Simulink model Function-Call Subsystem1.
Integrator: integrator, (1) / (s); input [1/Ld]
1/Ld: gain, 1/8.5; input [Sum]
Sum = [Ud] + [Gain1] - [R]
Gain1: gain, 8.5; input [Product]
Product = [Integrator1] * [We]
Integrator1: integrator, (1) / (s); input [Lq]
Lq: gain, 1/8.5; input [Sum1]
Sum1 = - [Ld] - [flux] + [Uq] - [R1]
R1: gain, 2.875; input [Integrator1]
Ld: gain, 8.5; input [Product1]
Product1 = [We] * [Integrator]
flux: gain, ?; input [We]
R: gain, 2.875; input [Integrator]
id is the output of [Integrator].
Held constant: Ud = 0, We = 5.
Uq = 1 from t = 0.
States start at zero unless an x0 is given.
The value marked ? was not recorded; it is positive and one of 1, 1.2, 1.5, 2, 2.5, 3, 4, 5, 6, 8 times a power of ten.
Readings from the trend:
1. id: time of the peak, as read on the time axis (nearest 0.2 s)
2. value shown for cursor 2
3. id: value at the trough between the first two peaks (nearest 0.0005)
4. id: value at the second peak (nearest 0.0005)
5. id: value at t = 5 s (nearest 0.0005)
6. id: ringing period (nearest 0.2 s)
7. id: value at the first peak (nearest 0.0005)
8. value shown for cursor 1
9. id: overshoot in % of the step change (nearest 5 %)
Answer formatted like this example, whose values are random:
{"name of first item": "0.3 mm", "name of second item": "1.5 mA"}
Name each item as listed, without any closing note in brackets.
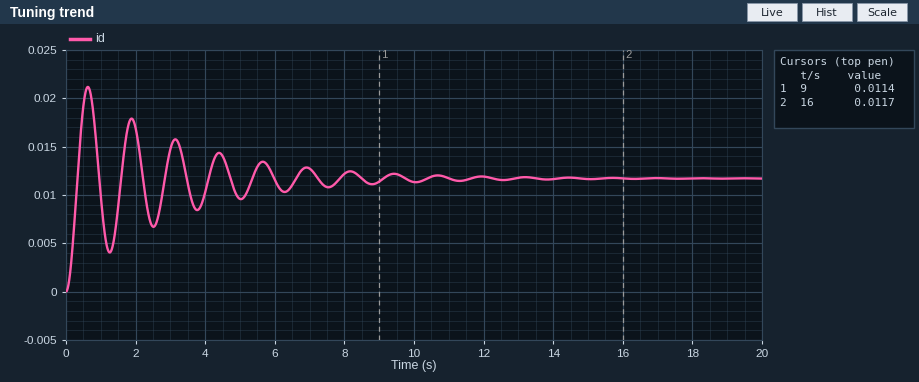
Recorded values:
{"id: time of the peak, as read on the time axis": "0.6 s", "value shown for cursor 2": "0.0117", "id: value at the trough between the first two peaks": "0.0040", "id: value at the second peak": "0.0180", "id: value at t = 5 s": "0.0095", "id: ringing period": "1.2 s", "id: value at the first peak": "0.0210", "value shown for cursor 1": "0.0114", "id: overshoot in % of the step change": "80 %"}
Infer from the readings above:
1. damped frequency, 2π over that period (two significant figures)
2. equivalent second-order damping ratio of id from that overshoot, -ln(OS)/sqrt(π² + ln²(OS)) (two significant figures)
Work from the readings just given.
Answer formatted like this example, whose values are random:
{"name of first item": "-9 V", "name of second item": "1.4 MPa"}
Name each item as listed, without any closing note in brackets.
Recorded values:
{"damped frequency, 2π over that period": "5.2 rad/s", "equivalent second-order damping ratio of id from that overshoot, -ln(OS)/sqrt(π² + ln²(OS))": "0.071"}
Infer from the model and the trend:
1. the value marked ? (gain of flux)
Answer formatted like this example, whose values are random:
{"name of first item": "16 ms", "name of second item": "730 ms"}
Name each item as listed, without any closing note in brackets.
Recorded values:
{"the value marked ?": "0.1"}
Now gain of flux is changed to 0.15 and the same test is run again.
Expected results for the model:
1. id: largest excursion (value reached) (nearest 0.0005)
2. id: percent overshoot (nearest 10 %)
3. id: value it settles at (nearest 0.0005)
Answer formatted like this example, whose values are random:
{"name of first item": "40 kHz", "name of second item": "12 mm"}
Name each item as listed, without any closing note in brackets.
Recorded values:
{"id: largest excursion (value reached)": "0.0105", "id: percent overshoot": "80 %", "id: value it settles at": "0.0060"}
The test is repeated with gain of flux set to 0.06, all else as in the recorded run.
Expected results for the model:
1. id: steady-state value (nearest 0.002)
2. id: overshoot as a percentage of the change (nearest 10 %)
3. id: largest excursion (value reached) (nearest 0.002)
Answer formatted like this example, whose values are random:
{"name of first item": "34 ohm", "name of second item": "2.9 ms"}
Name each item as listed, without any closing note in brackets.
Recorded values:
{"id: steady-state value": "0.016", "id: overshoot as a percentage of the change": "80 %", "id: largest excursion (value reached)": "0.030"}
